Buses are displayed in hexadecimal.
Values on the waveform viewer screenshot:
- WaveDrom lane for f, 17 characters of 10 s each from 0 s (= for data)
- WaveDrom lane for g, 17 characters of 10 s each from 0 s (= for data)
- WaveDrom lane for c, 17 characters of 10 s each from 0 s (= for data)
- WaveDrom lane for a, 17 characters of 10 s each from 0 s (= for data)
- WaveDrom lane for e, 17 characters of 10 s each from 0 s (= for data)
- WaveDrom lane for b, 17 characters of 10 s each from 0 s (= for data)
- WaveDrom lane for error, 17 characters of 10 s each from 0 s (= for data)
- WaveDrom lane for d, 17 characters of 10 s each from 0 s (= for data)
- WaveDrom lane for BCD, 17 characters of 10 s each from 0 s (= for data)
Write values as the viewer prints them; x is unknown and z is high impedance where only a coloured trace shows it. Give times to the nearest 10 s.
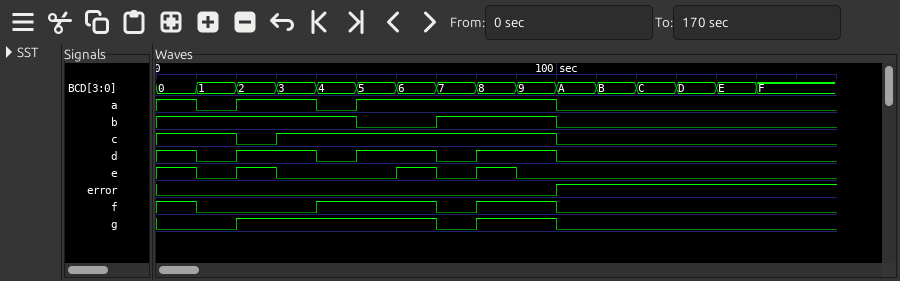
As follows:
{name: 'f', wave: '10..1..01.0......'}
{name: 'g', wave: '0.1....01.0......'}
{name: 'c', wave: '1.01......0......'}
{name: 'a', wave: '101.01....0......'}
{name: 'e', wave: '1010..1010.......'}
{name: 'b', wave: '1....0.1..0......'}
{name: 'error', wave: '0.........1......'}
{name: 'd', wave: '101.01.01.0......'}
{name: 'BCD', wave: '================.', data: '0 1 2 3 4 5 6 7 8 9 A B C D E F'}
